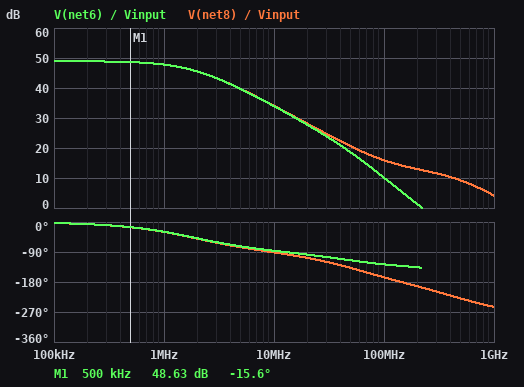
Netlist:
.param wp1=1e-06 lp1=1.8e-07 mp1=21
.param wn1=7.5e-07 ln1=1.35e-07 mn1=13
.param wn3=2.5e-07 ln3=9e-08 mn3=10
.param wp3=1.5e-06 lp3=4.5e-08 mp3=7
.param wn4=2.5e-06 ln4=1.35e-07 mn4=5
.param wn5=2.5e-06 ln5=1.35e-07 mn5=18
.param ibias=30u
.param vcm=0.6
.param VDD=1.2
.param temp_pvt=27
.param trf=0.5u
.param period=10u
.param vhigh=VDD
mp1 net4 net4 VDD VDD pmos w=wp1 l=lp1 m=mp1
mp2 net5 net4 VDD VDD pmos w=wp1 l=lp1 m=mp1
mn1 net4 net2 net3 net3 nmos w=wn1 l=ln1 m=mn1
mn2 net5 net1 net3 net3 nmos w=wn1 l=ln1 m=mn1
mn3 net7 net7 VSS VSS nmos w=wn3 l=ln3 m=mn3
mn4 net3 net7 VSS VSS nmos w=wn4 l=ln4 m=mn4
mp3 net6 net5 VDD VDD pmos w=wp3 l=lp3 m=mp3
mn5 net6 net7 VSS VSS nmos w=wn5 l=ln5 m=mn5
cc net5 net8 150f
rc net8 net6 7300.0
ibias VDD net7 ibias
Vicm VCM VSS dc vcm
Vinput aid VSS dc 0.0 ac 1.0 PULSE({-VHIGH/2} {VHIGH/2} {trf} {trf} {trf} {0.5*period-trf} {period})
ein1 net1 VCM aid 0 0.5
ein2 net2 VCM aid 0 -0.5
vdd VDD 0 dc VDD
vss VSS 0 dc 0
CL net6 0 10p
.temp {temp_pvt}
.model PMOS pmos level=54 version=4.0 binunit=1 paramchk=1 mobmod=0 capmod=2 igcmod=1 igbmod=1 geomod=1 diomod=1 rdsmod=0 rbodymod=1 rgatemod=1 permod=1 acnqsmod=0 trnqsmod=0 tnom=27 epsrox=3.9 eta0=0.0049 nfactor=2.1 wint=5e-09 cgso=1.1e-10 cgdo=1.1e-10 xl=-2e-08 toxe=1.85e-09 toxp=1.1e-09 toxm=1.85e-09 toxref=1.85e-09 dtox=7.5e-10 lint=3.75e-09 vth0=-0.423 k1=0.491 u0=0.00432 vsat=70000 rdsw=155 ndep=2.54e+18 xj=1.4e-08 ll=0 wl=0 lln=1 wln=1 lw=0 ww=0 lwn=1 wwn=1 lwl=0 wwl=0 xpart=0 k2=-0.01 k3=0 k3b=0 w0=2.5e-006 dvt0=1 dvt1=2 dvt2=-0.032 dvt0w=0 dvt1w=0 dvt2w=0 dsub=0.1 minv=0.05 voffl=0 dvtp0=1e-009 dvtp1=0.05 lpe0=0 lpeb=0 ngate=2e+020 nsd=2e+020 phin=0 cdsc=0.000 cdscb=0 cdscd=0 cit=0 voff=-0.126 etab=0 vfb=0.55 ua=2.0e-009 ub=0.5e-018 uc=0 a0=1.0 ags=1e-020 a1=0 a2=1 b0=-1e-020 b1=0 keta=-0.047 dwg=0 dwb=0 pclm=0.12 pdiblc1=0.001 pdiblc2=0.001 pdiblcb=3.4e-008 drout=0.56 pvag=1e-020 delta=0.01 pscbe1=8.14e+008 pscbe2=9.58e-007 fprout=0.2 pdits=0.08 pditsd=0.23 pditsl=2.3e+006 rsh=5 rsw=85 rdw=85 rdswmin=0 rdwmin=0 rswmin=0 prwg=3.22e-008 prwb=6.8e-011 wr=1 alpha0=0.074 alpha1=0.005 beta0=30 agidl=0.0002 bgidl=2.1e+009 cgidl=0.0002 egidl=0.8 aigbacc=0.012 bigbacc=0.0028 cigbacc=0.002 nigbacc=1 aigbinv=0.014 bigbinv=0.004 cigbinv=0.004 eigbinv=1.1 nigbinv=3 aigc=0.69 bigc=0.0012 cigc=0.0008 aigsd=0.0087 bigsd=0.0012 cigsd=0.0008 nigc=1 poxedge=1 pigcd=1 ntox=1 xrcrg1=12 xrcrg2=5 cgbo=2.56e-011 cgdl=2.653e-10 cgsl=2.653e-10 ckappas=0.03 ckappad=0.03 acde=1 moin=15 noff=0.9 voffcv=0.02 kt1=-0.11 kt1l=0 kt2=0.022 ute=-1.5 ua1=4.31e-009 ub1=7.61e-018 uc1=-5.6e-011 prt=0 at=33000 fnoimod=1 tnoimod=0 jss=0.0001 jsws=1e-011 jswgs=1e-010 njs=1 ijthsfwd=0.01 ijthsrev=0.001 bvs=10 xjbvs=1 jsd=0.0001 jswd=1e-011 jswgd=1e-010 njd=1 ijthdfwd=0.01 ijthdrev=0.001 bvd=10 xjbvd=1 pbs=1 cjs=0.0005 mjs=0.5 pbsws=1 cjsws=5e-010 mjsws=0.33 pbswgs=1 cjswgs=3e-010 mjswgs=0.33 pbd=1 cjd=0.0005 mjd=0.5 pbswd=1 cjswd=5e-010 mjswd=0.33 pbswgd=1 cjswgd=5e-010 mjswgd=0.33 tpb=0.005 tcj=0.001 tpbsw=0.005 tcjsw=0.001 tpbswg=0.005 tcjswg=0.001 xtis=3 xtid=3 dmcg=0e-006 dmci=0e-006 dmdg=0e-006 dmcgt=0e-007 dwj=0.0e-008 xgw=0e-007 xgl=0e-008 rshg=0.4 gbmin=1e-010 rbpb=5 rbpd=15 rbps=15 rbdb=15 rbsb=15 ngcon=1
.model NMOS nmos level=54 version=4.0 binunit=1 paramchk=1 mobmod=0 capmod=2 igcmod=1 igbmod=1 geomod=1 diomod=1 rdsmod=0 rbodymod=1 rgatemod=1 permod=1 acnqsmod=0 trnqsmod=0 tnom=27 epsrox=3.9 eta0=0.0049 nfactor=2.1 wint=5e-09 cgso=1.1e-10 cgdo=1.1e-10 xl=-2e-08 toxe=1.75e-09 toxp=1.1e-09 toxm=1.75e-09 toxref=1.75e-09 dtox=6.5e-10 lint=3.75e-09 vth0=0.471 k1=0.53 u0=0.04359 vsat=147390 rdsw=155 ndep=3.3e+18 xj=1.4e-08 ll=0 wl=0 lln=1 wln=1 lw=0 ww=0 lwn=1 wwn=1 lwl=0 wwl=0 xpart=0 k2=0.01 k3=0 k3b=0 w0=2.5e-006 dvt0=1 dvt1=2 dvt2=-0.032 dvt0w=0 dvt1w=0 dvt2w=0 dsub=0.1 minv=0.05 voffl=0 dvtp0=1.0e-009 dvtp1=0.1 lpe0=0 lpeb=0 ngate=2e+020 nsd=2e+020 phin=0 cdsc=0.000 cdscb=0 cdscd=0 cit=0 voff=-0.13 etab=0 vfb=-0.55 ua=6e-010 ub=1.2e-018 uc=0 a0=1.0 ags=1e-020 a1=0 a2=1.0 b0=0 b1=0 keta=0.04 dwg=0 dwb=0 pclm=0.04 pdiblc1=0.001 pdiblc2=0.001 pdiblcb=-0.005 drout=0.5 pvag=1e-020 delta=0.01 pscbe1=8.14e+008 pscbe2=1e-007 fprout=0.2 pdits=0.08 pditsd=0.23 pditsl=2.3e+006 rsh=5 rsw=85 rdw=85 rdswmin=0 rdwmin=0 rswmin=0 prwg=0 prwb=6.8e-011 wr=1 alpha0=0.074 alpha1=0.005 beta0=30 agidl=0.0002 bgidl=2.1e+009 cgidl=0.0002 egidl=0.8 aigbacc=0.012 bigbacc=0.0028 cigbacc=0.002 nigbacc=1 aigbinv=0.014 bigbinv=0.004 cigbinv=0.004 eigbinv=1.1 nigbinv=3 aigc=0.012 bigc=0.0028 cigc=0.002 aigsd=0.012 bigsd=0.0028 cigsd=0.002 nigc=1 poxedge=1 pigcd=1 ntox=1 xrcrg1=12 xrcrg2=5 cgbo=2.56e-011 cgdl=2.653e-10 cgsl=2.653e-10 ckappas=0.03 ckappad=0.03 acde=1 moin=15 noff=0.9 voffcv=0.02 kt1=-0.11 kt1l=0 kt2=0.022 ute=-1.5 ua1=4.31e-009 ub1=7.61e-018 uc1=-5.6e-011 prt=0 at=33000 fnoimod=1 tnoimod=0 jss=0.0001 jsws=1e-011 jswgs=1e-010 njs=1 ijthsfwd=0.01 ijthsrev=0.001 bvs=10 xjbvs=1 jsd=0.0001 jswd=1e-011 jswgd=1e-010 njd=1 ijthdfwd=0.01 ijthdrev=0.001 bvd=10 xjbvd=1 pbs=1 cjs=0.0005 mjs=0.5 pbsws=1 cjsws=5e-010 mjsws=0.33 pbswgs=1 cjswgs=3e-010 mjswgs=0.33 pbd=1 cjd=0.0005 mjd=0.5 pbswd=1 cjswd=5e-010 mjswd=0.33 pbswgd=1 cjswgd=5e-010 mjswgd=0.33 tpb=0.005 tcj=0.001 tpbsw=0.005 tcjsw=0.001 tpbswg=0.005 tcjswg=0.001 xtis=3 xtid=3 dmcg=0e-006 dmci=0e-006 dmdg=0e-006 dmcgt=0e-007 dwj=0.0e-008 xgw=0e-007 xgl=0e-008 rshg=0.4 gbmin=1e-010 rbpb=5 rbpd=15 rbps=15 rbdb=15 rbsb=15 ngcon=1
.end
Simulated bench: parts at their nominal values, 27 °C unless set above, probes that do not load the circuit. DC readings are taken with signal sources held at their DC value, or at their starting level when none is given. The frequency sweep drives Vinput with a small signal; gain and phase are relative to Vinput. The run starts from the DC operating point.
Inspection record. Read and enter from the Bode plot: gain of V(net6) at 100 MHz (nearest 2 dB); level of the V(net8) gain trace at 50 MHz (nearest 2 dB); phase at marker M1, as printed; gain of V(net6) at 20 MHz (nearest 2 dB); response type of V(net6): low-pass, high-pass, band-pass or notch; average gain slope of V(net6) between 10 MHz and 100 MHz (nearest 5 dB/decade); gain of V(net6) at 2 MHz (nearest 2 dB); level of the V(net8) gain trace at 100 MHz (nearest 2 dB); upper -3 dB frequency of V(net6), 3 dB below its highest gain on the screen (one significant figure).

10 dB
20 dB
-15.6 deg
28 dB
low-pass
-25 dB/decade
46 dB
16 dB
2 MHz
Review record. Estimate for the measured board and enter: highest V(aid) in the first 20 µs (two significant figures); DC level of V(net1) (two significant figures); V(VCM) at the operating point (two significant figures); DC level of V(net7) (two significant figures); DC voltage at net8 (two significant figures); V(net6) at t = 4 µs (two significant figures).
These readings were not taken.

600 mV
600 mV
600 mV
460 mV
960 mV
1.2 V
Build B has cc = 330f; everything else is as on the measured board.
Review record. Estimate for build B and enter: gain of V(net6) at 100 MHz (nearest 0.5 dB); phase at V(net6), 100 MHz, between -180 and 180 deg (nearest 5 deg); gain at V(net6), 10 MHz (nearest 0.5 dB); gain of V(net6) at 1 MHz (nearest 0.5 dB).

7.5 dB
-105 deg
28.0 dB
45.5 dB
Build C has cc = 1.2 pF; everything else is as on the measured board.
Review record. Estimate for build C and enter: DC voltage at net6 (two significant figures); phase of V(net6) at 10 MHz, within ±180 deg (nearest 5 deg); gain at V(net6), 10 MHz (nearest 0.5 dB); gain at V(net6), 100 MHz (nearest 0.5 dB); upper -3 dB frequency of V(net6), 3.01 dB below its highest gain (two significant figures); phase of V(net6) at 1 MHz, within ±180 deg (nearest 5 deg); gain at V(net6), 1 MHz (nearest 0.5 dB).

960 mV
-70 deg
18.5 dB
7.0 dB
270 kHz
-75 deg
37.0 dB
